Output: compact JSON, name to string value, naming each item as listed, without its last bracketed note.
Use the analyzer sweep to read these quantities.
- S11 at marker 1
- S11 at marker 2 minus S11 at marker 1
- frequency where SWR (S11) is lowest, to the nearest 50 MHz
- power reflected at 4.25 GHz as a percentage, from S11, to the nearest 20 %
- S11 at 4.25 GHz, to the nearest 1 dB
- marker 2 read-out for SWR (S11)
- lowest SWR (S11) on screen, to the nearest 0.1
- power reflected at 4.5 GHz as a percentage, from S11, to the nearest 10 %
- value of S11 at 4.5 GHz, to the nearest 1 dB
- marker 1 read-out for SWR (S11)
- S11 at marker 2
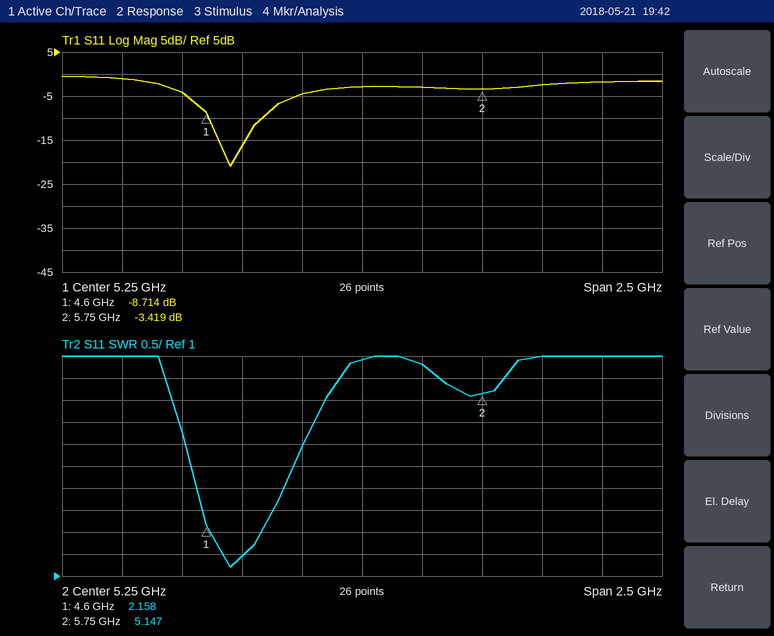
{"S11 at marker 1": "-8.714 dB", "S11 at marker 2 minus S11 at marker 1": "5.295 dB", "frequency where SWR (S11) is lowest, to the nearest 50 MHz": "4.70 GHz", "power reflected at 4.25 GHz as a percentage, from S11, to the nearest 20 %": "80 %", "S11 at 4.25 GHz, to the nearest 1 dB": "-1 dB", "marker 2 read-out for SWR": "5.147", "lowest SWR (S11) on screen, to the nearest 0.1": "1.2", "power reflected at 4.5 GHz as a percentage, from S11, to the nearest 10 %": "40 %", "value of S11 at 4.5 GHz, to the nearest 1 dB": "-4 dB", "marker 1 read-out for SWR": "2.158", "S11 at marker 2": "-3.419 dB"}
